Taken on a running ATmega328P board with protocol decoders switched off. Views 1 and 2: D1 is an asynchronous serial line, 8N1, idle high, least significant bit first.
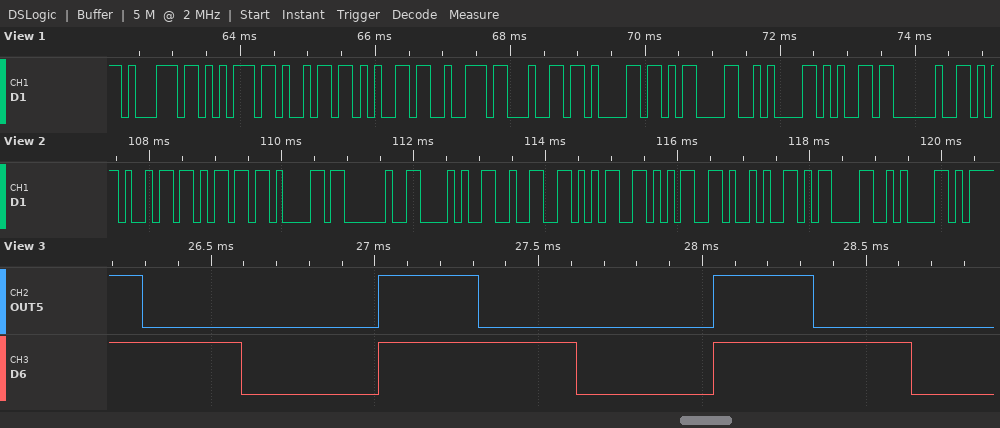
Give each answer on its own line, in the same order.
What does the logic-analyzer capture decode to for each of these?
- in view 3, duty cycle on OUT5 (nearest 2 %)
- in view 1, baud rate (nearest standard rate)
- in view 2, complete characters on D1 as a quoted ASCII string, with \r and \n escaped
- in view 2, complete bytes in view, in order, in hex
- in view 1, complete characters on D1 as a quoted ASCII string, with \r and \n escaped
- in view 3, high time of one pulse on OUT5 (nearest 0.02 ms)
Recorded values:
30 %
9600 baud
"ima (255)\r\n"
69 6D 61 20 28 32 35 35 29 0D 0A
"quierda\r\ne "
0.30 ms
